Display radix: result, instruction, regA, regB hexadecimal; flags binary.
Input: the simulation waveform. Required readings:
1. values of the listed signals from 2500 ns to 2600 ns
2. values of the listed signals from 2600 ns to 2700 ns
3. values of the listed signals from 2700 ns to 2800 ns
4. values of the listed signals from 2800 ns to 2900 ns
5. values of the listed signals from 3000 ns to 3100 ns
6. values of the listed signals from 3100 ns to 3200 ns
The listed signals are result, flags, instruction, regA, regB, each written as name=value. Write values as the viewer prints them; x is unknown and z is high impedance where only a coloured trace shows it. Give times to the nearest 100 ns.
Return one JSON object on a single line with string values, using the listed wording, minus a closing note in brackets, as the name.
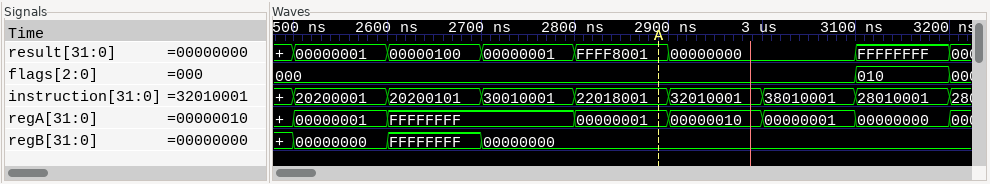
{"values of the listed signals from 2500 ns to 2600 ns": "result=00000001, flags=000, instruction=20200001, regA=00000001, regB=00000000", "values of the listed signals from 2600 ns to 2700 ns": "result=00000100, flags=000, instruction=20200101, regA=FFFFFFFF, regB=FFFFFFFF", "values of the listed signals from 2700 ns to 2800 ns": "result=00000001, flags=000, instruction=30010001, regA=FFFFFFFF, regB=00000000", "values of the listed signals from 2800 ns to 2900 ns": "result=FFFF8001, flags=000, instruction=22018001, regA=00000001, regB=00000000", "values of the listed signals from 3000 ns to 3100 ns": "result=00000000, flags=000, instruction=38010001, regA=00000001, regB=00000000", "values of the listed signals from 3100 ns to 3200 ns": "result=FFFFFFFF, flags=010, instruction=28010001, regA=00000000, regB=00000000"}
